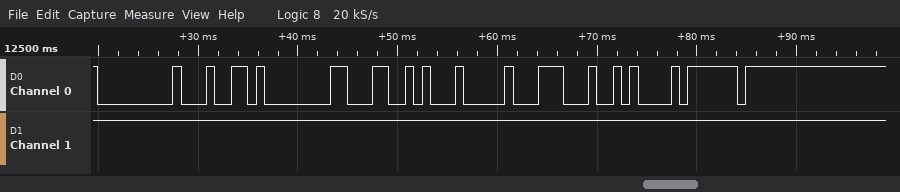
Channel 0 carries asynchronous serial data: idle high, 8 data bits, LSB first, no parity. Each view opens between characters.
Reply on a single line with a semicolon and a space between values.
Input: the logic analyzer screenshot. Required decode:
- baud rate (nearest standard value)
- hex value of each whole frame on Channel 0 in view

1200 baud; 00, 64, 80, 4C, 04, 1C, 0A, BF
